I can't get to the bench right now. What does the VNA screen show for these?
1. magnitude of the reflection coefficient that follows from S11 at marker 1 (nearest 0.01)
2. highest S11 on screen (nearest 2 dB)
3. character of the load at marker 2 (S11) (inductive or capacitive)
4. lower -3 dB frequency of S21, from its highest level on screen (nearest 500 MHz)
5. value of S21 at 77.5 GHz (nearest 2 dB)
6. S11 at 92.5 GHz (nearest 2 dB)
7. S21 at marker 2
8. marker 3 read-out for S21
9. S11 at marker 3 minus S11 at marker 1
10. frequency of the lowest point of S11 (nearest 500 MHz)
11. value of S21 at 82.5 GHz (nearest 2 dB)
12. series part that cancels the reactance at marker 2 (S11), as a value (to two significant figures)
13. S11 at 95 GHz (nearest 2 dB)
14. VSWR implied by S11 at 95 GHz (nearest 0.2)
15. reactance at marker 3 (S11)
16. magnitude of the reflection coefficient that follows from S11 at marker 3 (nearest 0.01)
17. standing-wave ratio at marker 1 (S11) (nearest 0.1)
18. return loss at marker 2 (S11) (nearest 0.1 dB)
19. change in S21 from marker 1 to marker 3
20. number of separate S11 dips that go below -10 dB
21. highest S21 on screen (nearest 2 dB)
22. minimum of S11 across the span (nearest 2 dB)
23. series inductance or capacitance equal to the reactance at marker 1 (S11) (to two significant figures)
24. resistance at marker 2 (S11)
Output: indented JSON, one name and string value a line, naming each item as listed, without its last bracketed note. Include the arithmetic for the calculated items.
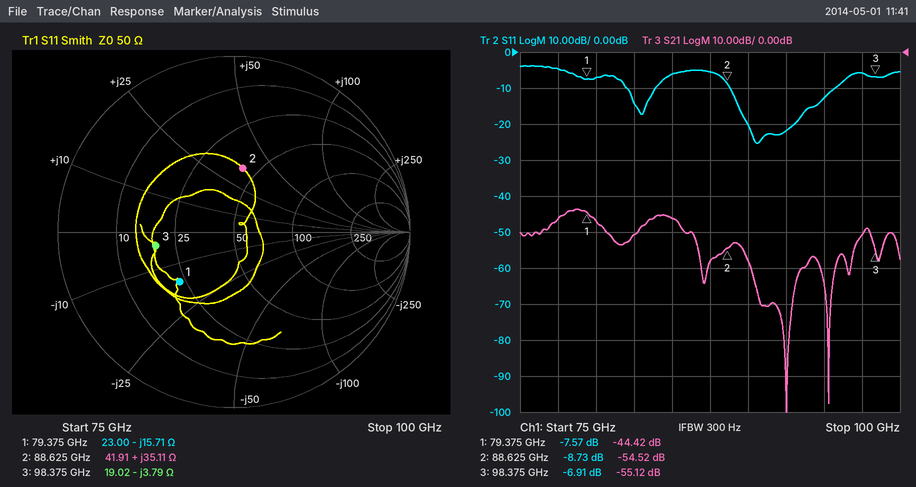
{
  "magnitude of the reflection coefficient that follows from S11 at marker 1": "10^(-7.57/20) ≈ 0.42",
  "highest S11 on screen": "-4 dB",
  "character of the load at marker 2 (S11)": "inductive",
  "lower -3 dB frequency of S21, from its highest level on screen": "77.5 GHz",
  "value of S21 at 77.5 GHz": "-46 dB",
  "S11 at 92.5 GHz": "-22 dB",
  "S21 at marker 2": "-54.52 dB",
  "marker 3 read-out for S21": "-55.12 dB",
  "S11 at marker 3 minus S11 at marker 1": "-6.91 − (-7.57) = 0.66 dB",
  "frequency of the lowest point of S11": "90.5 GHz",
  "value of S21 at 82.5 GHz": "-50 dB",
  "series part that cancels the reactance at marker 2 (S11), as a value": "C = 1/(2π × 88.625 GHz × 35.11 Ω) ≈ 51 fF",
  "S11 at 95 GHz": "-12 dB",
  "VSWR implied by S11 at 95 GHz": "|Γ| = 10^(-12/20) = 0.2512; VSWR = (1 + 0.2512)/(1 − 0.2512) ≈ 1.67, so 1.6 to the nearest 0.2",
  "reactance at marker 3": "-3.79 Ω",
  "magnitude of the reflection coefficient that follows from S11 at marker 3": "10^(-6.91/20) ≈ 0.45",
  "standing-wave ratio at marker 1 (S11)": "2.4",
  "return loss at marker 2 (S11)": "8.7 dB",
  "change in S21 from marker 1 to marker 3": "-55.12 − (-44.42) = -10.70 dB",
  "number of separate S11 dips that go below -10 dB": "2",
  "highest S21 on screen": "-44 dB",
  "minimum of S11 across the span": "-26 dB",
  "series inductance or capacitance equal to the reactance at marker 1 (S11)": "C = 1/(2π × 79.375 GHz × 15.71 Ω) ≈ 128 fF, so 130 fF to two significant figures",
  "resistance at marker 2": "41.91 Ω"
}
